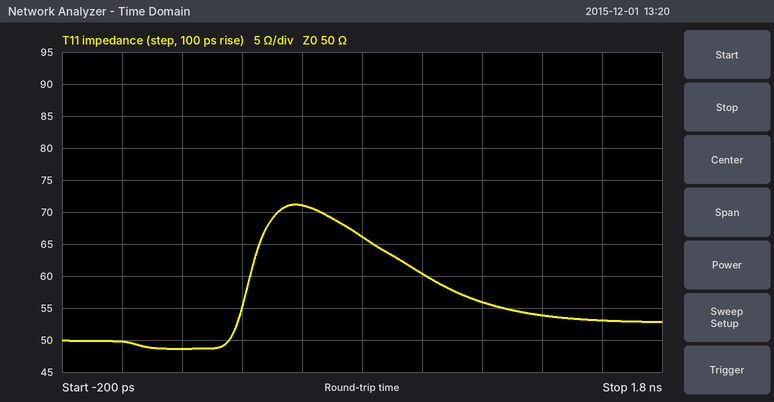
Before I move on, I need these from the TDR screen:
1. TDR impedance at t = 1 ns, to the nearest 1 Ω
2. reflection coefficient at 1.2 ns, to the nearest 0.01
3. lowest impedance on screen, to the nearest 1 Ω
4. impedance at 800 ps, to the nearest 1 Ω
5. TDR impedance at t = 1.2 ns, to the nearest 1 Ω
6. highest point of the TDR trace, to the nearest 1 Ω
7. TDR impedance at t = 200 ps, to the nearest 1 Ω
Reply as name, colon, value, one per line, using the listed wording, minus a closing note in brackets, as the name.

TDR impedance at t = 1 ns, to the nearest 1 Ω: 60 Ω
reflection coefficient at 1.2 ns, to the nearest 0.01: +0.06
lowest impedance on screen, to the nearest 1 Ω: 49 Ω
impedance at 800 ps, to the nearest 1 Ω: 66 Ω
TDR impedance at t = 1.2 ns, to the nearest 1 Ω: 56 Ω
highest point of the TDR trace, to the nearest 1 Ω: 71 Ω
TDR impedance at t = 200 ps, to the nearest 1 Ω: 49 Ω
